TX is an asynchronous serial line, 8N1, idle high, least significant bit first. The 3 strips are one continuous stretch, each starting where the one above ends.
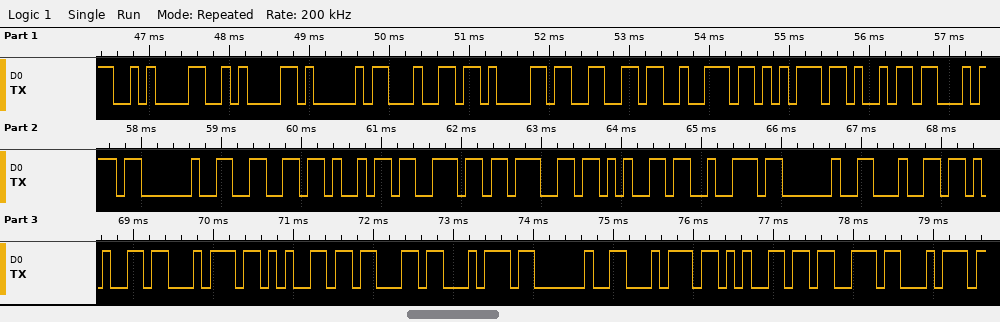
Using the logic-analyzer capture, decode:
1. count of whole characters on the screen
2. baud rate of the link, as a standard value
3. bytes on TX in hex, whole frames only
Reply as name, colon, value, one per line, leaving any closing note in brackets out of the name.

count of whole characters on the screen: 29
baud rate of the link, as a standard value: 9600 baud
bytes on TX in hex, whole frames only: 0x0A 0x0A 0x41 0x64 0x61 0x66 0x72 0x75 0x69 0x74 0x20 0x66 0x69 0x6E 0x67 0x65 0x72 0x20 0x64 0x65 0x74 0x65 0x63 0x74 0x20 0x74 0x65 0x73 0x74
